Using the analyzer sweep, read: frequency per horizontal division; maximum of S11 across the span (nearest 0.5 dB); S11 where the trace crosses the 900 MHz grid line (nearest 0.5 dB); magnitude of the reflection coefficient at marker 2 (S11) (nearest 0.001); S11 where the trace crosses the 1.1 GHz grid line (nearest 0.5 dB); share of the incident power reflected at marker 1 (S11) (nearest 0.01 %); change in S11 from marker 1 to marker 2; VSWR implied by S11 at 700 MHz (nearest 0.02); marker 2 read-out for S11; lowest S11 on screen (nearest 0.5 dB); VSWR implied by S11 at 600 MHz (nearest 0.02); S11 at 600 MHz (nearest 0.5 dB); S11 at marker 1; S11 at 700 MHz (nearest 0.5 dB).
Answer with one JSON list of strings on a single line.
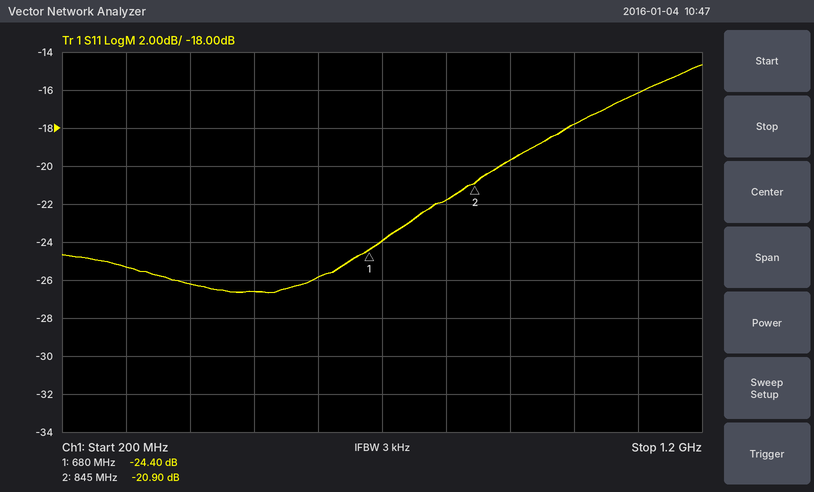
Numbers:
["100 MHz", "-14.5 dB", "-19.5 dB", "0.090", "-16.0 dB", "0.36 %", "3.50 dB", "1.14", "-20.90 dB", "-26.5 dB", "1.10", "-26.0 dB", "-24.40 dB", "-24.0 dB"]
